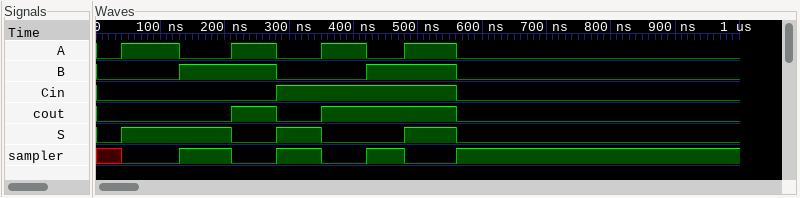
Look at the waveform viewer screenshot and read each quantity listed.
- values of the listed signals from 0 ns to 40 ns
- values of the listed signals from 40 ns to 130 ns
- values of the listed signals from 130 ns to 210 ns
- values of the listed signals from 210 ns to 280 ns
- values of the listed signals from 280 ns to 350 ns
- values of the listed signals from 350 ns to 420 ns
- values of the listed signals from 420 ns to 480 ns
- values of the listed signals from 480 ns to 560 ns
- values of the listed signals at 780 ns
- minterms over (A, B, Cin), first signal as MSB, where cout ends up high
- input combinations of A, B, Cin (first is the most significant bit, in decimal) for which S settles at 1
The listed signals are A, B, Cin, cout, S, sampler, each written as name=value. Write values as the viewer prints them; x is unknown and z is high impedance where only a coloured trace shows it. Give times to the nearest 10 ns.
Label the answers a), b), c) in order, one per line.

a) A=0, B=0, Cin=0, cout=0, S=0, sampler=x
b) A=1, B=0, Cin=0, cout=0, S=1, sampler=0
c) A=0, B=1, Cin=0, cout=0, S=1, sampler=1
d) A=1, B=1, Cin=0, cout=1, S=0, sampler=0
e) A=0, B=0, Cin=1, cout=0, S=1, sampler=1
f) A=1, B=0, Cin=1, cout=1, S=0, sampler=0
g) A=0, B=1, Cin=1, cout=1, S=0, sampler=1
h) A=1, B=1, Cin=1, cout=1, S=1, sampler=0
i) A=0, B=0, Cin=0, cout=0, S=0, sampler=1
j) 3, 5, 6, 7
k) 1, 2, 4, 7
